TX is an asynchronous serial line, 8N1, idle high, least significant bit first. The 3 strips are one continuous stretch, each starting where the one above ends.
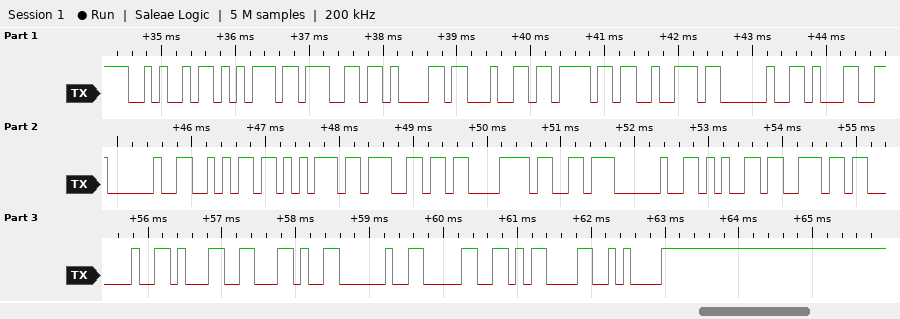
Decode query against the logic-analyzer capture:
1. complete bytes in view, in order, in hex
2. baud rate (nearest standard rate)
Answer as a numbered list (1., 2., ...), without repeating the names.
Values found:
1. 4A 75 67 61 64 6F 72 20 31 20 6A 75 67 C3 B3 20 65 6E 20 31 2C 20 30 0D 0A
2. 9600 baud
